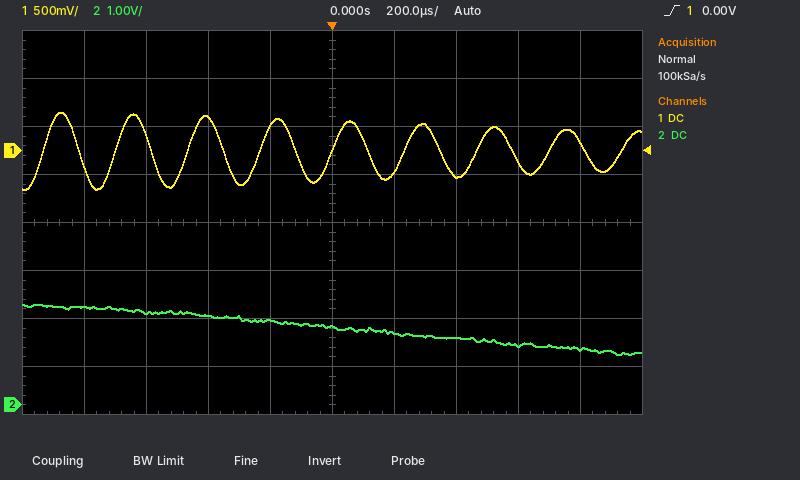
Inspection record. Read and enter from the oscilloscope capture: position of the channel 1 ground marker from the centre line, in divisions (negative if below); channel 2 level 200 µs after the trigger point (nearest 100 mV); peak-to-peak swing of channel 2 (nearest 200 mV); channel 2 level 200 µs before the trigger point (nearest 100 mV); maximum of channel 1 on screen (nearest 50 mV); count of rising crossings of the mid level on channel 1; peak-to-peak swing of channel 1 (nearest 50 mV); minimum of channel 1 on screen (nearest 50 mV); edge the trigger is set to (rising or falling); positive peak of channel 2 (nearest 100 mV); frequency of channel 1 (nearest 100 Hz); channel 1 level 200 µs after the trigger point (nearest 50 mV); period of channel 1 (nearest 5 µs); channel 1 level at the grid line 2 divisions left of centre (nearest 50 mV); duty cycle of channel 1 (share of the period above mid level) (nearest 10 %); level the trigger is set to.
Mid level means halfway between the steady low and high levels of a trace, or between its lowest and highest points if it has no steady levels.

+1.5 div
1.5 V
1.0 V
1.8 V
400 mV
9
800 mV
-400 mV
rising
2.1 V
4.3 kHz
-200 mV
235 µs
350 mV
50 %
0.00 V
